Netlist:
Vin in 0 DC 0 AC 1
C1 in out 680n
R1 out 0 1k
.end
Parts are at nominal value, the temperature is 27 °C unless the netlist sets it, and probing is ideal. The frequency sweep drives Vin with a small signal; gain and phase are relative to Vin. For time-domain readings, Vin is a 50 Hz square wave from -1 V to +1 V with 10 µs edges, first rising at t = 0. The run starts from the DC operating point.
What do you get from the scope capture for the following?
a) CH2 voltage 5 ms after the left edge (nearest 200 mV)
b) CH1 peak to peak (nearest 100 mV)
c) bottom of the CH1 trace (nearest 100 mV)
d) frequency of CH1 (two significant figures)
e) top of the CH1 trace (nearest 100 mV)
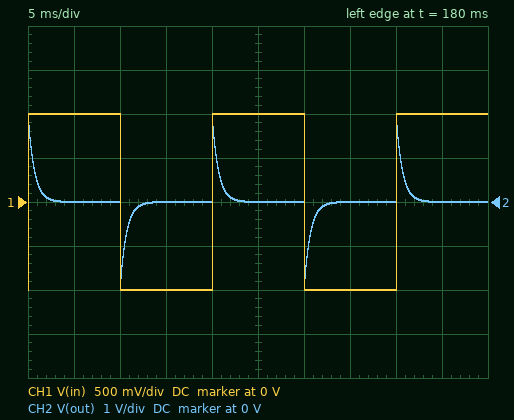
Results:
0 V
2.0 V
-1.0 V
50 Hz
1.0 V
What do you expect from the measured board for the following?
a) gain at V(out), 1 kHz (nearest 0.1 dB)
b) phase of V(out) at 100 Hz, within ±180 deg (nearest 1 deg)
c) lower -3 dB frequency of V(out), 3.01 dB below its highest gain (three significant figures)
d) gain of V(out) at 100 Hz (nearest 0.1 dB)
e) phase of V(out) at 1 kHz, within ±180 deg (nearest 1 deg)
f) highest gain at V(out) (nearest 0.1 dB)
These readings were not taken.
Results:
-0.2 dB
67 deg
234 Hz
-8.1 dB
13 deg
0 dB
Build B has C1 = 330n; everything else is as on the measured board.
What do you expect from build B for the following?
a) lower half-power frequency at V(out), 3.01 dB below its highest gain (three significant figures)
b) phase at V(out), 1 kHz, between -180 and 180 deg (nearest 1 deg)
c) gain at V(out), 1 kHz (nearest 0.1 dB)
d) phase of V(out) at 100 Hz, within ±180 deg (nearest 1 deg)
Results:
482 Hz
26 deg
-0.9 dB
78 deg
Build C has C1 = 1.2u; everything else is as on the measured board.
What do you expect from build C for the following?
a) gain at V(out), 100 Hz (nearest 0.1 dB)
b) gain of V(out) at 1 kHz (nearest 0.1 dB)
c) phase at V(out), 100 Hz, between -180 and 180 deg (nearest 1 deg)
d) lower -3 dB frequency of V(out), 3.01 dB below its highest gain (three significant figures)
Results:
-4.4 dB
-0.1 dB
53 deg
133 Hz
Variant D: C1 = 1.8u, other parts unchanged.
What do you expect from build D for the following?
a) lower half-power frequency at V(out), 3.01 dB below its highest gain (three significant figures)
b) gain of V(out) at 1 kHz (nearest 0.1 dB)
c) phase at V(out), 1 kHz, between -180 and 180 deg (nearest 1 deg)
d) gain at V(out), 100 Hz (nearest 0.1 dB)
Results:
88.4 Hz
0 dB
5 deg
-2.5 dB
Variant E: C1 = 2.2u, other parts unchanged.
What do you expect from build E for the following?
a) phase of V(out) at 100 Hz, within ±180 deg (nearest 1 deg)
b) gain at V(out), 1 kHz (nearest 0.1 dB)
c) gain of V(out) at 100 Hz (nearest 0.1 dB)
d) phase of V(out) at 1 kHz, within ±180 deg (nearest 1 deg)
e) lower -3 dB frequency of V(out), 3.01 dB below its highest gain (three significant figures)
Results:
36 deg
0 dB
-1.8 dB
4 deg
72.3 Hz
